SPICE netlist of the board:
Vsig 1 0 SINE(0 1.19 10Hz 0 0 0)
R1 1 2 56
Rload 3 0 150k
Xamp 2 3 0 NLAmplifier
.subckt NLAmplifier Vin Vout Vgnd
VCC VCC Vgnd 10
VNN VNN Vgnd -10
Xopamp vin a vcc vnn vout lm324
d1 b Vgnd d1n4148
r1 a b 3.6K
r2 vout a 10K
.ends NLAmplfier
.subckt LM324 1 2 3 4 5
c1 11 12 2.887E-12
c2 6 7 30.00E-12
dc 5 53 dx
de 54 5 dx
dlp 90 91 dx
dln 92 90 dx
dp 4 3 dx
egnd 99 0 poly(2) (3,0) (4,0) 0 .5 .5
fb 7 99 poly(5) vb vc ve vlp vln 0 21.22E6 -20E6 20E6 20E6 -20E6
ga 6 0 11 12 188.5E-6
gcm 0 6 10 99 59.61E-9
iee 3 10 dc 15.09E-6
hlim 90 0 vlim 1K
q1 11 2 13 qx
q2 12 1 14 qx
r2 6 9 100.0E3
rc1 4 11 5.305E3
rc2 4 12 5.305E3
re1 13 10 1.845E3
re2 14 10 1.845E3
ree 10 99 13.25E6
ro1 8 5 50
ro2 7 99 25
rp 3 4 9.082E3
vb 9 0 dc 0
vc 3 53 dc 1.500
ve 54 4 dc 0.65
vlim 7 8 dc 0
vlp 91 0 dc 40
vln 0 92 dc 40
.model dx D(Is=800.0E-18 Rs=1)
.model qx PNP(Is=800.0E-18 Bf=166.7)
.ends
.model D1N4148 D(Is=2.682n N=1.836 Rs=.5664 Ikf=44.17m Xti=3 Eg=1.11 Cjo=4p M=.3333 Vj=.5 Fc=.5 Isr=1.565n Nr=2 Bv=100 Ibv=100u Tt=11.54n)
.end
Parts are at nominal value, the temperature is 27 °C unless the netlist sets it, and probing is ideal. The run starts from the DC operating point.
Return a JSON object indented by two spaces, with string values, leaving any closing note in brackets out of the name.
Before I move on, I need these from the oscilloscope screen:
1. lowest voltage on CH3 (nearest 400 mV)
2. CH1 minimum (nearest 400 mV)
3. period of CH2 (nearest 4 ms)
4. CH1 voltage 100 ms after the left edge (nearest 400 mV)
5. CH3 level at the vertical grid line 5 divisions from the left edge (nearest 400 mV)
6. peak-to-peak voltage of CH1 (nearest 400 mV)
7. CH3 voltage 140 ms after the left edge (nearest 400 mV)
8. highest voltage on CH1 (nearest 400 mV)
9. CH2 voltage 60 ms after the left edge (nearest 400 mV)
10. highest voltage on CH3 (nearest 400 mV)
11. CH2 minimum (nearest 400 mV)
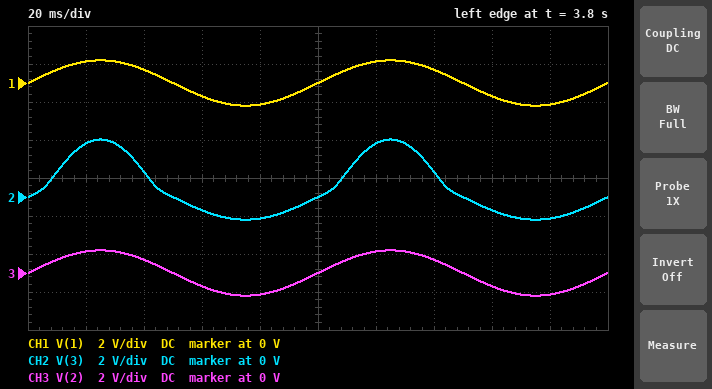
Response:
{
  "lowest voltage on CH3": "-1.2 V",
  "CH1 minimum": "-1.2 V",
  "period of CH2": "100 ms",
  "CH1 voltage 100 ms after the left edge": "0 V",
  "CH3 level at the vertical grid line 5 divisions from the left edge": "0 V",
  "peak-to-peak voltage of CH1": "2.4 V",
  "CH3 voltage 140 ms after the left edge": "800 mV",
  "highest voltage on CH1": "1.2 V",
  "CH2 voltage 60 ms after the left edge": "-800 mV",
  "highest voltage on CH3": "1.2 V",
  "CH2 minimum": "-1.2 V"
}
